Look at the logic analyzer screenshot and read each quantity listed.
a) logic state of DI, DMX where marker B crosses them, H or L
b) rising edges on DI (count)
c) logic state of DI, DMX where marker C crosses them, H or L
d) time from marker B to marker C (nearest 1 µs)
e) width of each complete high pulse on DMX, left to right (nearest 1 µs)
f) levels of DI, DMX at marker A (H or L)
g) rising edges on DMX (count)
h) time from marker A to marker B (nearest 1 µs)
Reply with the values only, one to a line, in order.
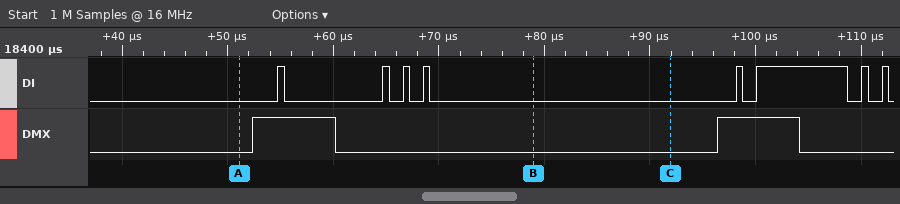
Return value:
DI=L, DMX=L
8
DI=L, DMX=L
13 µs
8 µs, 8 µs
DI=L, DMX=L
2
28 µs
